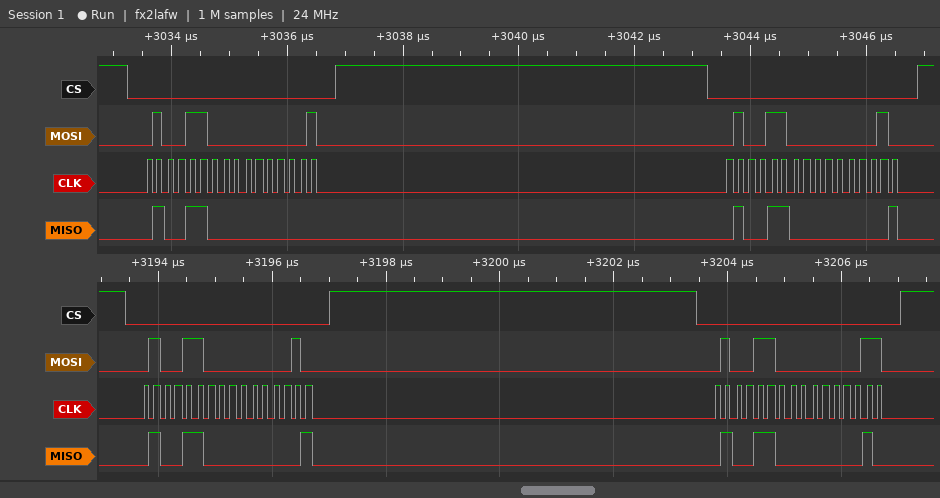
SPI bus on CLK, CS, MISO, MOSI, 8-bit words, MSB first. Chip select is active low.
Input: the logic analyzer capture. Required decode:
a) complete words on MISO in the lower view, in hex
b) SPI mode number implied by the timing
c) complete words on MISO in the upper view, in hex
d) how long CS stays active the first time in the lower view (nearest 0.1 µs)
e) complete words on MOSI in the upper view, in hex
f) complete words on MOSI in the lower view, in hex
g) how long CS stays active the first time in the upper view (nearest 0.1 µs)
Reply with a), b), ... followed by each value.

a) 4C, 01, 4C, 02
b) 0
c) 4C, 00, 4C, 01
d) 3.6 µs
e) 4C, 01, 4C, 02
f) 4C, 02, 4C, 03
g) 3.6 µs
